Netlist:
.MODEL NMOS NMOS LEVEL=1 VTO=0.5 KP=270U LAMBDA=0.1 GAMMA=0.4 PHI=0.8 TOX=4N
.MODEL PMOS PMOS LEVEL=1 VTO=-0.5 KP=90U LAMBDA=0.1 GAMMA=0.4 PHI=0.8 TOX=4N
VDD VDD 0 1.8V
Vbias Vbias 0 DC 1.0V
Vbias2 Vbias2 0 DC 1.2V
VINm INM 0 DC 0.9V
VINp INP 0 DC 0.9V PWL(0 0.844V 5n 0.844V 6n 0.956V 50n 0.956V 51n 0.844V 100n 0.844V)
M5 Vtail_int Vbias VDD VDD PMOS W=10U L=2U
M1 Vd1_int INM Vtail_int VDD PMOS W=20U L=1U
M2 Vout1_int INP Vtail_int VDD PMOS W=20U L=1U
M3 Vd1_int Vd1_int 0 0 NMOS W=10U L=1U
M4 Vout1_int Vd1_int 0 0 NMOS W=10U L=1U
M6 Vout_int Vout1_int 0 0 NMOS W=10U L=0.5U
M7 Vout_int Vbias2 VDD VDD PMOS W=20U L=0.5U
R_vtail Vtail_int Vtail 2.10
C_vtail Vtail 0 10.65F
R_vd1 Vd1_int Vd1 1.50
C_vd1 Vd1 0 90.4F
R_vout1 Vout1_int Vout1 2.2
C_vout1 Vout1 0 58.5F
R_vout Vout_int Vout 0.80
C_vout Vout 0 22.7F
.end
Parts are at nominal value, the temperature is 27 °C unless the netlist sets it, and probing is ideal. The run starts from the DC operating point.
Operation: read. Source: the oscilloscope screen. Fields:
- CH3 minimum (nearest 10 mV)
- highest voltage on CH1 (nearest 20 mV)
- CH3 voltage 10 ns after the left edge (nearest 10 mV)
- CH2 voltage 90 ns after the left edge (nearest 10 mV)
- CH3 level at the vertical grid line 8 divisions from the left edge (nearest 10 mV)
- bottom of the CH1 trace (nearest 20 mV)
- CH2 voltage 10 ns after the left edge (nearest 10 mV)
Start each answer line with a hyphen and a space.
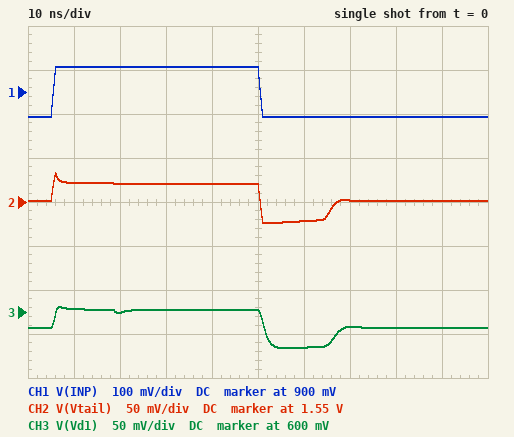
- 560 mV
- 960 mV
- 600 mV
- 1.55 V
- 580 mV
- 840 mV
- 1.57 V
